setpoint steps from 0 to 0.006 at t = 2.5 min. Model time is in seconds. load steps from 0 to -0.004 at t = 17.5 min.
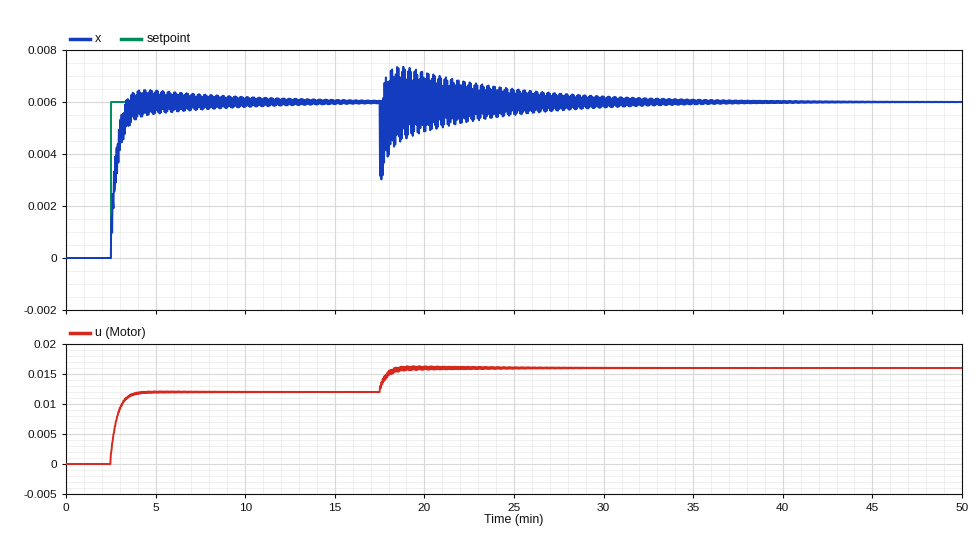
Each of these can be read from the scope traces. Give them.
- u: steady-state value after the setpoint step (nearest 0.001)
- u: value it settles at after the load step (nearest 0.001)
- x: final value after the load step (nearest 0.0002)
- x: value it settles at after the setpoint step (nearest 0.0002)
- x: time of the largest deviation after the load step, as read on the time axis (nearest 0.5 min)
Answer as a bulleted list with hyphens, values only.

- 0.012
- 0.016
- 0.0060
- 0.0060
- 17.5 min
